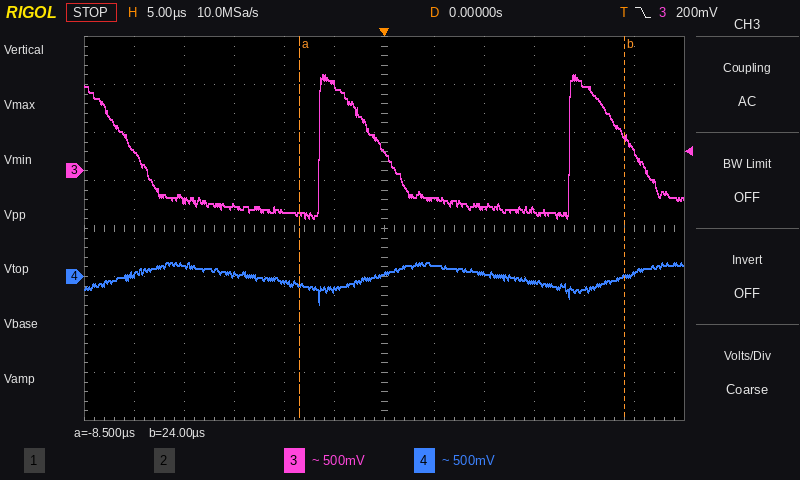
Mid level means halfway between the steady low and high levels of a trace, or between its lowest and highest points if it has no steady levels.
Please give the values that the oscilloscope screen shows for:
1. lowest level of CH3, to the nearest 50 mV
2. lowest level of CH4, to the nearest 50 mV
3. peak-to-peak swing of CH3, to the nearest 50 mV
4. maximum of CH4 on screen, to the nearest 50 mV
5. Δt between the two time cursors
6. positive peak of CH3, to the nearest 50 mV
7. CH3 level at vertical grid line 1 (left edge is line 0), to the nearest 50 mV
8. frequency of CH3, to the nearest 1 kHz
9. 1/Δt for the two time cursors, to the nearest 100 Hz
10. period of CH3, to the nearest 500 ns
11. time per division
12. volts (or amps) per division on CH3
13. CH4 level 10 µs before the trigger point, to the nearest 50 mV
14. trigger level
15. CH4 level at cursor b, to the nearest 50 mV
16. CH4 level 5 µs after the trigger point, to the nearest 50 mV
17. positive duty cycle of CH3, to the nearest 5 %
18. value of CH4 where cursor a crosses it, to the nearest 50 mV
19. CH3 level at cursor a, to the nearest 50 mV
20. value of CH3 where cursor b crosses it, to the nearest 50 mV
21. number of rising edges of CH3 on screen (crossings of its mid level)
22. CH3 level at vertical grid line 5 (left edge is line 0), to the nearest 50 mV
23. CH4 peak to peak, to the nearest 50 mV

-500 mV
-300 mV
1.50 V
150 mV
32.5 µs
1.00 V
200 mV
40 kHz
30.8 kHz
25.0 µs
5 µs
500 mV
-50 mV
200 mV
0 mV
100 mV
25 %
-100 mV
-450 mV
350 mV
2
900 mV
450 mV
